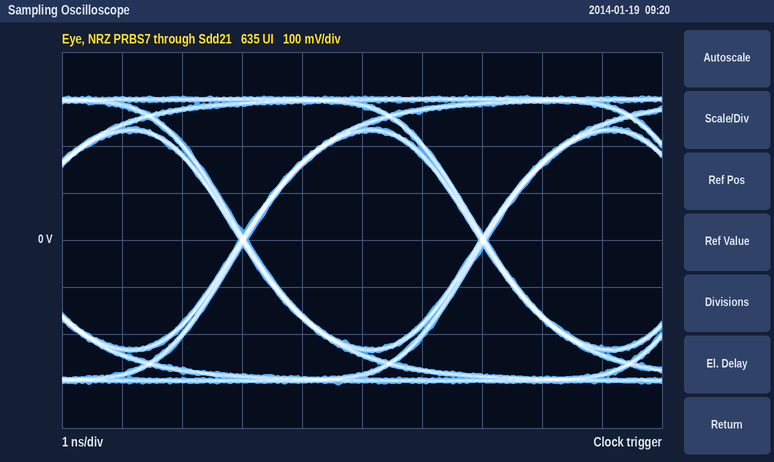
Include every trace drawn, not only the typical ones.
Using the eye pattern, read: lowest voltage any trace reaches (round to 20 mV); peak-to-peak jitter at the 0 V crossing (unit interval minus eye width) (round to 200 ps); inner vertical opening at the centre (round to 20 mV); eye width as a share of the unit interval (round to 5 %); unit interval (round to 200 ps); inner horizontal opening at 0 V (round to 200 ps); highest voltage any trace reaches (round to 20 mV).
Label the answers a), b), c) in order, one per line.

a) -300 mV
b) 200 ps
c) 460 mV
d) 95 %
e) 4.0 ns
f) 3.8 ns
g) 300 mV
